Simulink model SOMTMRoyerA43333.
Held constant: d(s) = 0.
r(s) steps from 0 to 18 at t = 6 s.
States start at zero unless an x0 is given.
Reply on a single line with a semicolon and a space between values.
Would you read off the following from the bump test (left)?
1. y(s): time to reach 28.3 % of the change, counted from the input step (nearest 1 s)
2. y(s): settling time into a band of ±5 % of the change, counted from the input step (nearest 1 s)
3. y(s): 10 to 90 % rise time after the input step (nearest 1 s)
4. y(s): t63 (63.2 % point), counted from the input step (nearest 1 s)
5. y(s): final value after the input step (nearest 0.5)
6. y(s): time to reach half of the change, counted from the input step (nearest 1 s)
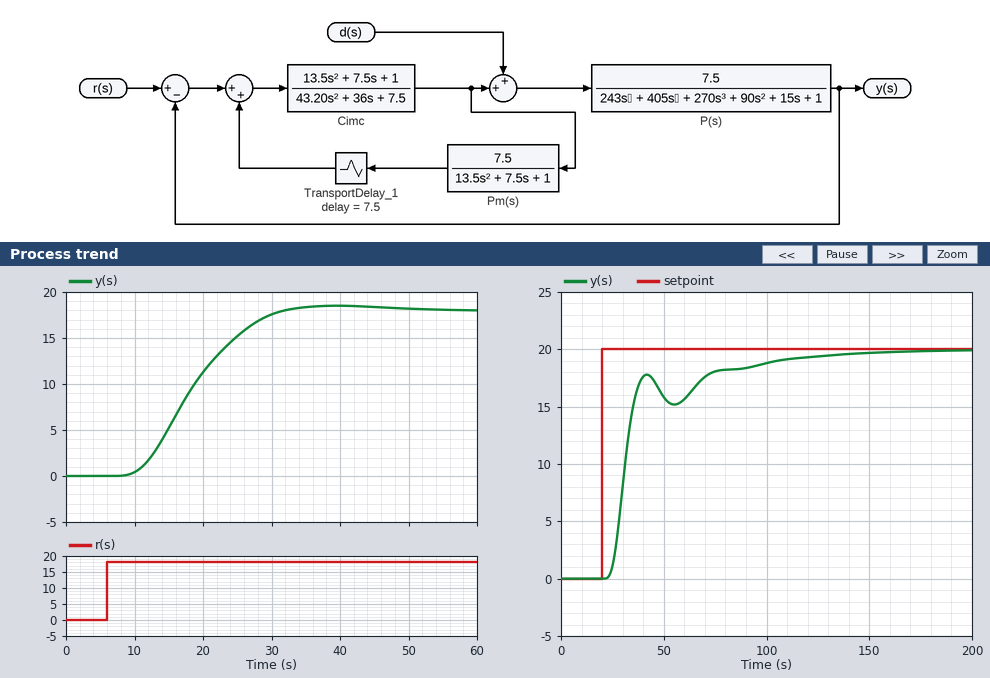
9 s; 23 s; 15 s; 14 s; 18.0; 12 s
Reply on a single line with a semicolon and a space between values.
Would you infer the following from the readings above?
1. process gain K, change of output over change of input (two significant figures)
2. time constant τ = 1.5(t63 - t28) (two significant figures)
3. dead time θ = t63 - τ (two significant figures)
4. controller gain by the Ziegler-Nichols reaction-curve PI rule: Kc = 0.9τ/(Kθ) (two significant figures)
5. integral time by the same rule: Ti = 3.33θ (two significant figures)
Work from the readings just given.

1.0; 7.5 s; 6.5 s; 1.0; 22 s
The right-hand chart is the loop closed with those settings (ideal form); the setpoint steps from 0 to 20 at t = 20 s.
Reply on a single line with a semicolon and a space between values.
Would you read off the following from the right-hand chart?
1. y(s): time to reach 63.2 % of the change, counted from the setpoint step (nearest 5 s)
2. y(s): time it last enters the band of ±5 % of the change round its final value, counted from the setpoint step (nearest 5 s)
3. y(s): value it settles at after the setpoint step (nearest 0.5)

15 s; 85 s; 20.0
